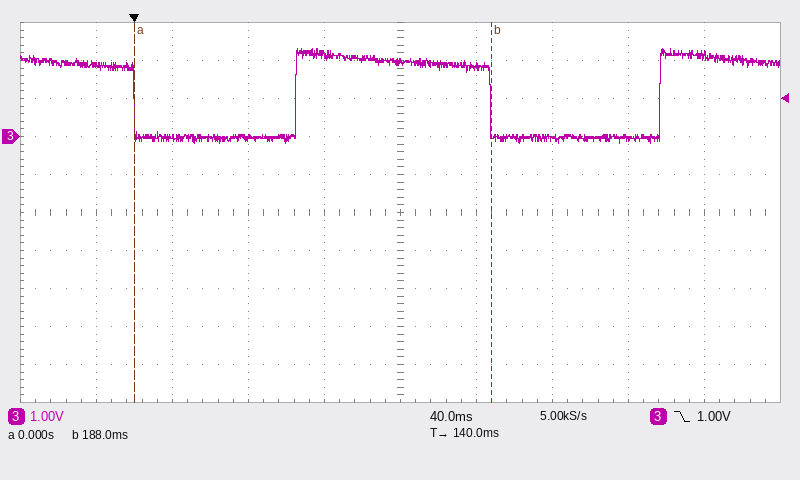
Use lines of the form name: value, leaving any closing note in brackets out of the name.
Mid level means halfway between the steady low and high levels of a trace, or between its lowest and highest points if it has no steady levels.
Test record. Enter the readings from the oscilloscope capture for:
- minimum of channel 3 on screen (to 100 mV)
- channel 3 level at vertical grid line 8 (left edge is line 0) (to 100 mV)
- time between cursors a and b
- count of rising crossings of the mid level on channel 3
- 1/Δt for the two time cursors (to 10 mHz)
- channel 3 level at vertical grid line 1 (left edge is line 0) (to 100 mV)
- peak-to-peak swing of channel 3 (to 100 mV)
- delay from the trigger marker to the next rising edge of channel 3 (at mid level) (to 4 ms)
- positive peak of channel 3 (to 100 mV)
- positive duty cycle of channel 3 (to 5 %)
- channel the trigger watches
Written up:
minimum of channel 3 on screen: -200 mV
channel 3 level at vertical grid line 8 (left edge is line 0): 0.0 V
time between cursors a and b: 188 ms
count of rising crossings of the mid level on channel 3: 2
1/Δt for the two time cursors: 5.32 Hz
channel 3 level at vertical grid line 1 (left edge is line 0): 1.9 V
peak-to-peak swing of channel 3: 2.5 V
delay from the trigger marker to the next rising edge of channel 3 (at mid level): 84 ms
positive peak of channel 3: 2.3 V
positive duty cycle of channel 3: 55 %
channel the trigger watches: channel 3
